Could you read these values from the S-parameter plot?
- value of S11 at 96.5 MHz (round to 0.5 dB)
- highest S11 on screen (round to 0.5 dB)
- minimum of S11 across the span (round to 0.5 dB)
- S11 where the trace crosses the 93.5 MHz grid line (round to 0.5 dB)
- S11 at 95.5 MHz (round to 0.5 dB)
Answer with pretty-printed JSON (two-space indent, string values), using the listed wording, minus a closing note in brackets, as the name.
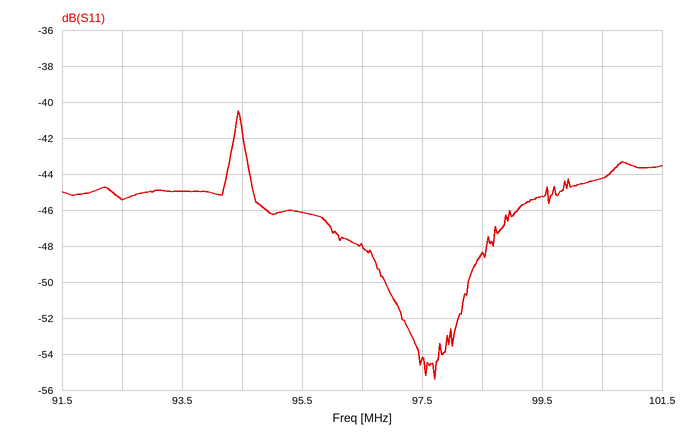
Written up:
{
  "value of S11 at 96.5 MHz": "-48.0 dB",
  "highest S11 on screen": "-40.5 dB",
  "minimum of S11 across the span": "-55.5 dB",
  "S11 where the trace crosses the 93.5 MHz grid line": "-45.0 dB",
  "S11 at 95.5 MHz": "-46.0 dB"
}
